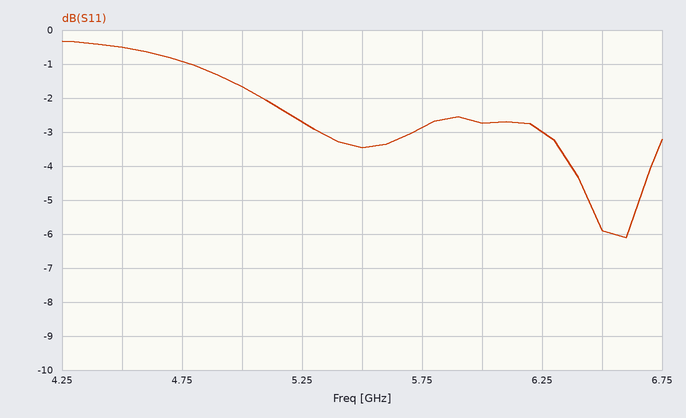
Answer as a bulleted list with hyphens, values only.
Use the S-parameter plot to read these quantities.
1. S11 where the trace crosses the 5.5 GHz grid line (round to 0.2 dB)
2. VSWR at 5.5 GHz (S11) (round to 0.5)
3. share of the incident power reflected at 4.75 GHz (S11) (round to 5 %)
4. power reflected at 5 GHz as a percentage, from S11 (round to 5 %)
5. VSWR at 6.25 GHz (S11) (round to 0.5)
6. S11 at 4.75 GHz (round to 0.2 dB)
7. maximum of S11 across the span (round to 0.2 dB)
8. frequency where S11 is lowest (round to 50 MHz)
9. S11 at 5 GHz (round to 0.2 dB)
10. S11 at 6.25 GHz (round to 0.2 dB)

- -3.4 dB
- 5.0
- 80 %
- 70 %
- 6.0
- -1.0 dB
- -0.4 dB
- 6.60 GHz
- -1.6 dB
- -3.0 dB
